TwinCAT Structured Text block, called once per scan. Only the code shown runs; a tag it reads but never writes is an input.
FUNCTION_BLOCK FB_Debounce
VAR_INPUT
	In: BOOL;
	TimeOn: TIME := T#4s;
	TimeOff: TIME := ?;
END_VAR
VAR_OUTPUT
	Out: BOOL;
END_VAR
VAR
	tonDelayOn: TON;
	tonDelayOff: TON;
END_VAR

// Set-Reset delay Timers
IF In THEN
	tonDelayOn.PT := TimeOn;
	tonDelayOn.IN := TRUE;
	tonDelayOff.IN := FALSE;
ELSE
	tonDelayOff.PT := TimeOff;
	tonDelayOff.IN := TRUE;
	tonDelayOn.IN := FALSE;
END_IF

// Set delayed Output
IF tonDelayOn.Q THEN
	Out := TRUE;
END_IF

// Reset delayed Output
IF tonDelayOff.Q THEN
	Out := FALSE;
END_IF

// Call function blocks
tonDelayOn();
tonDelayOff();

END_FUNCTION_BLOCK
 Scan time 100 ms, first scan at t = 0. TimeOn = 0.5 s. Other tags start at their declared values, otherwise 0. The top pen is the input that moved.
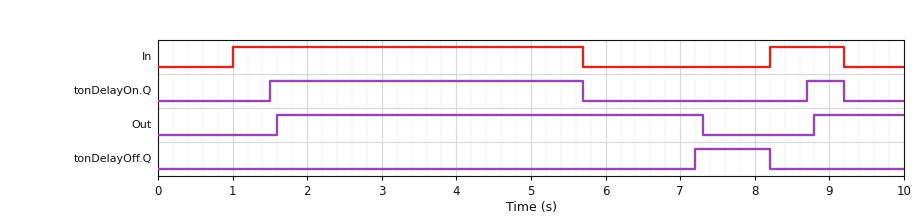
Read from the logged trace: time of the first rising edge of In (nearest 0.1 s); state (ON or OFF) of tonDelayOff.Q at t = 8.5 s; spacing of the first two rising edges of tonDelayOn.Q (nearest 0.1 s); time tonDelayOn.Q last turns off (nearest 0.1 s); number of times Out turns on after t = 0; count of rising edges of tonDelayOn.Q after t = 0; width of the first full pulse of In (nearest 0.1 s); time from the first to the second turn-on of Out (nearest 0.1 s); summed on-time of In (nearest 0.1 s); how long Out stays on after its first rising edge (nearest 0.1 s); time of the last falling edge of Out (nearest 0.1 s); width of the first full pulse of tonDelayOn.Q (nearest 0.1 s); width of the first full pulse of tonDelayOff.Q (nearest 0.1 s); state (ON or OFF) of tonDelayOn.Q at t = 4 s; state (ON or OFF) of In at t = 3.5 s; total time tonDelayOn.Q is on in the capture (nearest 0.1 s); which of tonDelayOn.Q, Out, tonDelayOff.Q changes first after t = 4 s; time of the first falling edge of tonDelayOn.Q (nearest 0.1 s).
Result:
1.0 s
OFF
7.2 s
9.2 s
2
2
4.7 s
7.2 s
5.7 s
5.7 s
7.3 s
4.2 s
1.0 s
ON
ON
4.7 s
tonDelayOn.Q
5.7 s
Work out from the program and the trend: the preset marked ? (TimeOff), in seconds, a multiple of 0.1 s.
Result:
1.5 s
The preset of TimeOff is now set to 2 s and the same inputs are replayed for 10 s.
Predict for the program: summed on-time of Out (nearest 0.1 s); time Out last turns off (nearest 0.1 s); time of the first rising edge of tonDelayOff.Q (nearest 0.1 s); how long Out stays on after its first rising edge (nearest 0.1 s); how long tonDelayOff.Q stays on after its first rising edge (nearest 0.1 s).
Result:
7.4 s
7.8 s
7.7 s
6.2 s
0.5 s
